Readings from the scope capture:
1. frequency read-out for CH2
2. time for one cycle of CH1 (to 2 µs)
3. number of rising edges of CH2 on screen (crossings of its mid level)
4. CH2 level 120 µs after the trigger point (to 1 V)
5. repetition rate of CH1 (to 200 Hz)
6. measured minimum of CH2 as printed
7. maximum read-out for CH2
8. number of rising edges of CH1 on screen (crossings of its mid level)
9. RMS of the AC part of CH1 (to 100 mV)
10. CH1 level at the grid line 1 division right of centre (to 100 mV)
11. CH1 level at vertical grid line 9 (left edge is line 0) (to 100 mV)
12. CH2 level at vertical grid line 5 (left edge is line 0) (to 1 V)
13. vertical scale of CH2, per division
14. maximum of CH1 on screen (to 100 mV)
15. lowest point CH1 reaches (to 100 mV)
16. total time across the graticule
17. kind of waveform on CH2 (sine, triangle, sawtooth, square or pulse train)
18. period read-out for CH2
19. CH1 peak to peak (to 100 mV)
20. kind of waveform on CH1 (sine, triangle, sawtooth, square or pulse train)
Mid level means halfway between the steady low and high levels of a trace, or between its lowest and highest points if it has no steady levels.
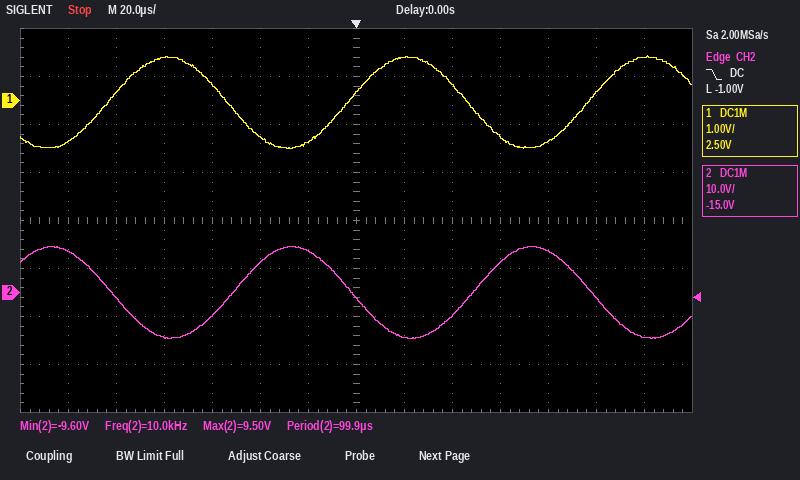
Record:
10.0 kHz
100 µs
2
-9 V
10.0 kHz
-9.60 V
9.50 V
3
700 mV
900 mV
300 mV
6 V
10 V
900 mV
-1.0 V
280 µs
sine
99.9 µs
1.9 V
sine
